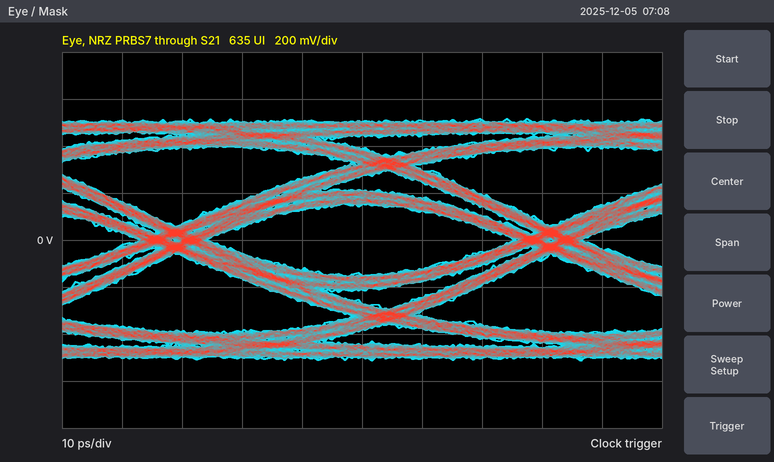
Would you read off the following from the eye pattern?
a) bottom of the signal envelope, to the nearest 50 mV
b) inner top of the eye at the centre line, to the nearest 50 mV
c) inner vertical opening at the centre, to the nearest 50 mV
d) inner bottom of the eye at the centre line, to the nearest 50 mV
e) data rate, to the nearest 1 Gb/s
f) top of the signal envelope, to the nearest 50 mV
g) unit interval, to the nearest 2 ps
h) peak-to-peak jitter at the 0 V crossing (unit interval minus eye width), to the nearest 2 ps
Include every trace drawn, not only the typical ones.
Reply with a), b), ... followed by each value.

a) -500 mV
b) 150 mV
c) 300 mV
d) -150 mV
e) 16 Gb/s
f) 500 mV
g) 62 ps
h) 12 ps
